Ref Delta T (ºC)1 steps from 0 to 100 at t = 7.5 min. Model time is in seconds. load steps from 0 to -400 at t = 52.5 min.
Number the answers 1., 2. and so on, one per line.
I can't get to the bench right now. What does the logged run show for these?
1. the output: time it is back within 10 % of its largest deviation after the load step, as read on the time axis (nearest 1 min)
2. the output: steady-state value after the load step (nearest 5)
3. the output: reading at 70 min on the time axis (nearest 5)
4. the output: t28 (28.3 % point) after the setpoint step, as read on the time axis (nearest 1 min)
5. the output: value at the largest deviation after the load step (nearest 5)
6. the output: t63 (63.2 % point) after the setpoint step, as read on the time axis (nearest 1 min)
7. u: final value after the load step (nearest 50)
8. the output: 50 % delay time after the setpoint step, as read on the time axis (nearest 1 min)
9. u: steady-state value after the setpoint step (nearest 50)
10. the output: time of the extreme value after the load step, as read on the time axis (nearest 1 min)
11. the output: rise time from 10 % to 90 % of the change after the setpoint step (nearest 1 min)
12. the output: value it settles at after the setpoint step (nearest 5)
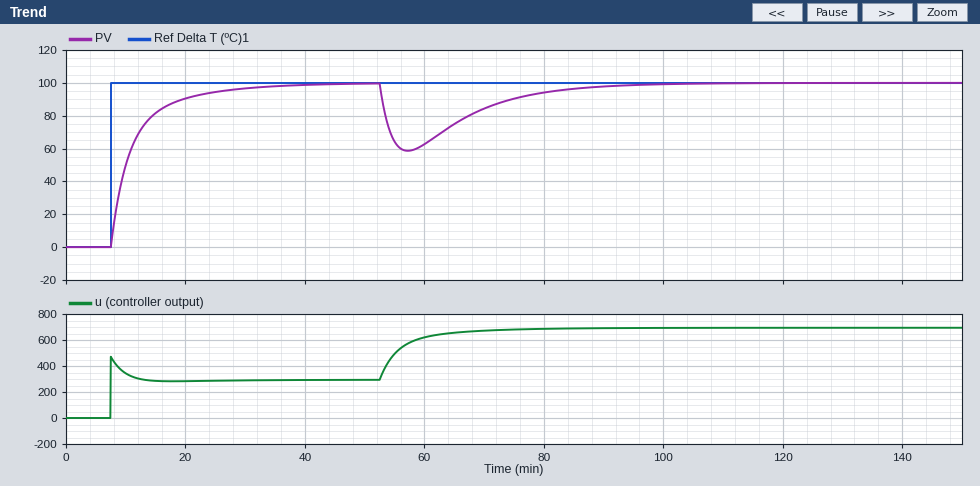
1. 84 min
2. 100
3. 85
4. 9 min
5. 60
6. 11 min
7. 700
8. 10 min
9. 300
10. 57 min
11. 12 min
12. 100
